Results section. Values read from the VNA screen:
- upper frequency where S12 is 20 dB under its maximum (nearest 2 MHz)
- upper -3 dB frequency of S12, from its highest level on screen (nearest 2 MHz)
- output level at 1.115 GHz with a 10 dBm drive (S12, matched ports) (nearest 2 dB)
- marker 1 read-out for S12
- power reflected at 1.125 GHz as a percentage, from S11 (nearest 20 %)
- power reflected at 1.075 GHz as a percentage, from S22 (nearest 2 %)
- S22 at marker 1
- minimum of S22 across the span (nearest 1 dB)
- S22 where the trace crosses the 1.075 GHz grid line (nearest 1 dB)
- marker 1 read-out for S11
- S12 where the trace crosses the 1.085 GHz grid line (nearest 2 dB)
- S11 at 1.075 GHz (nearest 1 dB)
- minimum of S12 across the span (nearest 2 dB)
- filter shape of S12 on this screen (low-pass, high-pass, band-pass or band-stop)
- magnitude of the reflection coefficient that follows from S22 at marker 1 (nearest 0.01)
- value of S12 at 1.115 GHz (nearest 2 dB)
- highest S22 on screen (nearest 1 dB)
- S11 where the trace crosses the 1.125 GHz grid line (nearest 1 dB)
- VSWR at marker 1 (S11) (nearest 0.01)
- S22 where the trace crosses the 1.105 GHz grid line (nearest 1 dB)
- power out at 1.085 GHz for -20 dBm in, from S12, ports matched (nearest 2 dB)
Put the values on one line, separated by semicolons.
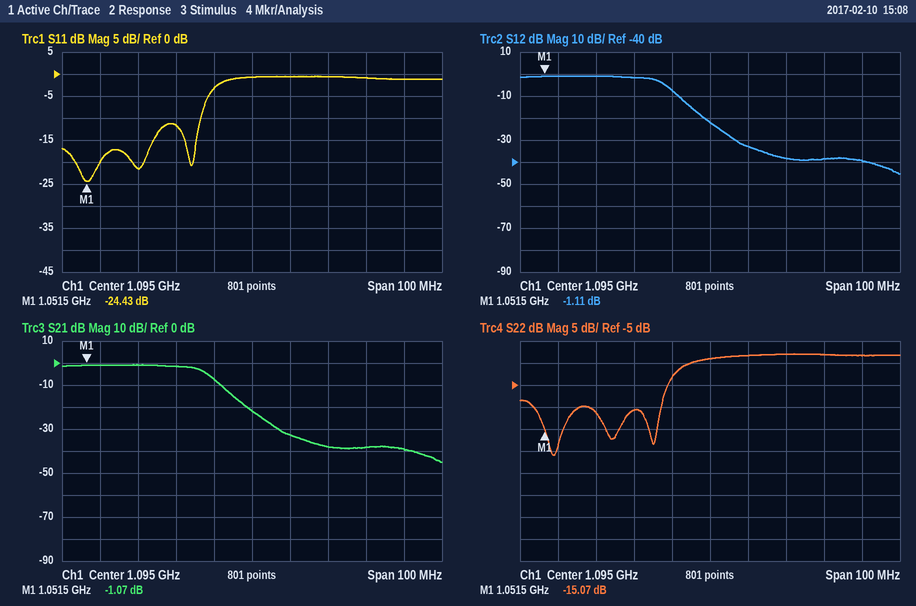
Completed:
1.094 GHz; 1.082 GHz; -28 dBm; -1.11 dB; 80 %; 8 %; -15.07 dB; -21 dB; -11 dB; -24.43 dB; -8 dB; -12 dB; -46 dB; low-pass; 0.18; -38 dB; 2 dB; -1 dB; 1.13; 2 dB; -28 dBm
